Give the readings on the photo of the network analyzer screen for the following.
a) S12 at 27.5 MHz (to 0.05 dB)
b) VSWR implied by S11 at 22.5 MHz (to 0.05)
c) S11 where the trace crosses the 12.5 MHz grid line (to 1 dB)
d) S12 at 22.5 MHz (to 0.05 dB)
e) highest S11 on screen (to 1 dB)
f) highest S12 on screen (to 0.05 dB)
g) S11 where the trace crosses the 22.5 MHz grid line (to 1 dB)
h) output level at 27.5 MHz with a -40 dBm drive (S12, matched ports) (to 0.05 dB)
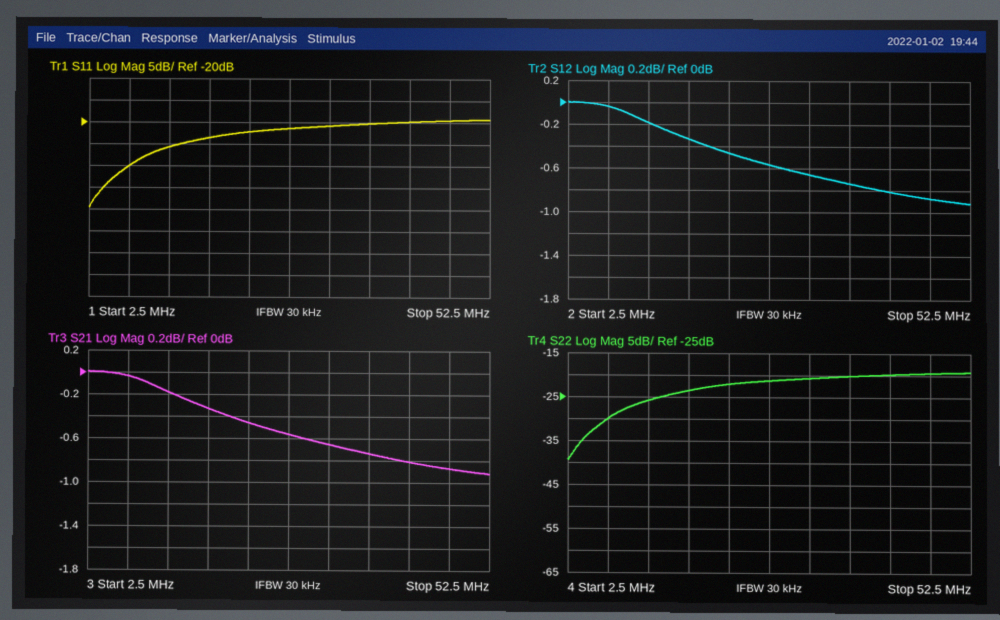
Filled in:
-0.55 dB
1.15
-26 dB
-0.45 dB
-19 dB
0.00 dB
-22 dB
-40.55 dBm
